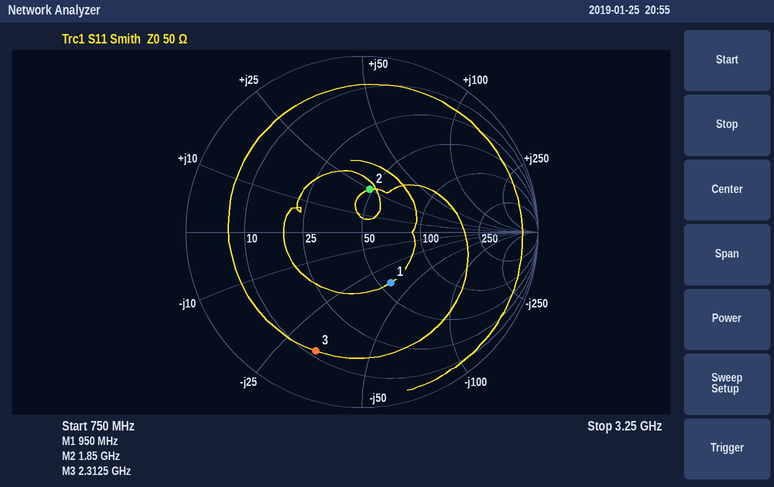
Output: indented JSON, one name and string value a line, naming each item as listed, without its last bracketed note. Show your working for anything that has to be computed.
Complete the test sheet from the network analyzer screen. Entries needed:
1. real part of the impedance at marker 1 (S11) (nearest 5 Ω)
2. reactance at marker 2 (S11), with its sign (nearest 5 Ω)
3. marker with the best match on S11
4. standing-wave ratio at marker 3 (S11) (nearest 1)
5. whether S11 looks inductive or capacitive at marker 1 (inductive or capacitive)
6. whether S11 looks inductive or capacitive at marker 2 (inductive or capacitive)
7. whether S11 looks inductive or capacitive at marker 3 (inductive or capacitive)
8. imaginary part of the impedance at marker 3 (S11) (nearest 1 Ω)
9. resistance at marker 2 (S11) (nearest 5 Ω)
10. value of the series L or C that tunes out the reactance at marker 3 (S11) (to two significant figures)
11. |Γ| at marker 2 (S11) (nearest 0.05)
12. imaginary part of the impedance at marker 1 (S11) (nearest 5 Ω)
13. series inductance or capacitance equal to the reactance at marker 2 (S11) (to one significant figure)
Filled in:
{
  "real part of the impedance at marker 1 (S11)": "55 Ω",
  "reactance at marker 2 (S11), with its sign": "+25 Ω",
  "marker with the best match on S11": "marker 2",
  "standing-wave ratio at marker 3 (S11)": "6",
  "whether S11 looks inductive or capacitive at marker 1": "capacitive",
  "whether S11 looks inductive or capacitive at marker 2": "inductive",
  "whether S11 looks inductive or capacitive at marker 3": "capacitive",
  "imaginary part of the impedance at marker 3 (S11)": "-33 Ω",
  "resistance at marker 2 (S11)": "50 Ω",
  "value of the series L or C that tunes out the reactance at marker 3 (S11)": "L = 33 Ω/(2π × 2.3125 GHz) ≈ 2.3 nH",
  "|Γ| at marker 2 (S11)": "0.25",
  "imaginary part of the impedance at marker 1 (S11)": "-35 Ω",
  "series inductance or capacitance equal to the reactance at marker 2 (S11)": "L = 25 Ω/(2π × 1.85 GHz) ≈ 2 nH"
}
